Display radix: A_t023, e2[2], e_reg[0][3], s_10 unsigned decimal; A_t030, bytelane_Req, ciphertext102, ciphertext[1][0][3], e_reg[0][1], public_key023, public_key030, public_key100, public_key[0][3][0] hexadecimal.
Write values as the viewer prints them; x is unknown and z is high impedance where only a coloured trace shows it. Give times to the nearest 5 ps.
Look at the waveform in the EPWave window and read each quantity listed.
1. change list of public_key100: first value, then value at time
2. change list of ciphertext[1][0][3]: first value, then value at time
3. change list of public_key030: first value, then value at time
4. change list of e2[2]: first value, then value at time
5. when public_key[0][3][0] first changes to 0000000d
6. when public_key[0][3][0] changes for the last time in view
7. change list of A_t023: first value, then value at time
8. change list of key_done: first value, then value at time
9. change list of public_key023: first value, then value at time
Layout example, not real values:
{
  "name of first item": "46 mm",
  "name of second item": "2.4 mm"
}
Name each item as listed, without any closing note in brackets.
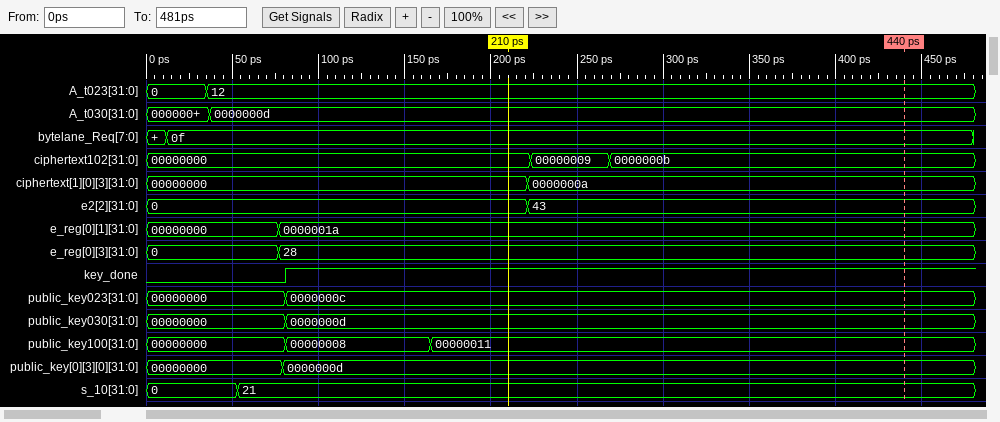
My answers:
{
  "change list of public_key100: first value, then value at time": "00000000, 00000008 at 80 ps, 00000011 at 165 ps",
  "change list of ciphertext[1][0][3]: first value, then value at time": "00000000, 0000000a at 220 ps",
  "change list of public_key030: first value, then value at time": "00000000, 0000000d at 80 ps",
  "change list of e2[2]: first value, then value at time": "0, 43 at 220 ps",
  "when public_key[0][3][0] first changes to 0000000d": "80 ps",
  "when public_key[0][3][0] changes for the last time in view": "80 ps",
  "change list of A_t023: first value, then value at time": "0, 12 at 35 ps",
  "change list of key_done: first value, then value at time": "0, 1 at 80 ps",
  "change list of public_key023: first value, then value at time": "00000000, 0000000c at 80 ps"
}
